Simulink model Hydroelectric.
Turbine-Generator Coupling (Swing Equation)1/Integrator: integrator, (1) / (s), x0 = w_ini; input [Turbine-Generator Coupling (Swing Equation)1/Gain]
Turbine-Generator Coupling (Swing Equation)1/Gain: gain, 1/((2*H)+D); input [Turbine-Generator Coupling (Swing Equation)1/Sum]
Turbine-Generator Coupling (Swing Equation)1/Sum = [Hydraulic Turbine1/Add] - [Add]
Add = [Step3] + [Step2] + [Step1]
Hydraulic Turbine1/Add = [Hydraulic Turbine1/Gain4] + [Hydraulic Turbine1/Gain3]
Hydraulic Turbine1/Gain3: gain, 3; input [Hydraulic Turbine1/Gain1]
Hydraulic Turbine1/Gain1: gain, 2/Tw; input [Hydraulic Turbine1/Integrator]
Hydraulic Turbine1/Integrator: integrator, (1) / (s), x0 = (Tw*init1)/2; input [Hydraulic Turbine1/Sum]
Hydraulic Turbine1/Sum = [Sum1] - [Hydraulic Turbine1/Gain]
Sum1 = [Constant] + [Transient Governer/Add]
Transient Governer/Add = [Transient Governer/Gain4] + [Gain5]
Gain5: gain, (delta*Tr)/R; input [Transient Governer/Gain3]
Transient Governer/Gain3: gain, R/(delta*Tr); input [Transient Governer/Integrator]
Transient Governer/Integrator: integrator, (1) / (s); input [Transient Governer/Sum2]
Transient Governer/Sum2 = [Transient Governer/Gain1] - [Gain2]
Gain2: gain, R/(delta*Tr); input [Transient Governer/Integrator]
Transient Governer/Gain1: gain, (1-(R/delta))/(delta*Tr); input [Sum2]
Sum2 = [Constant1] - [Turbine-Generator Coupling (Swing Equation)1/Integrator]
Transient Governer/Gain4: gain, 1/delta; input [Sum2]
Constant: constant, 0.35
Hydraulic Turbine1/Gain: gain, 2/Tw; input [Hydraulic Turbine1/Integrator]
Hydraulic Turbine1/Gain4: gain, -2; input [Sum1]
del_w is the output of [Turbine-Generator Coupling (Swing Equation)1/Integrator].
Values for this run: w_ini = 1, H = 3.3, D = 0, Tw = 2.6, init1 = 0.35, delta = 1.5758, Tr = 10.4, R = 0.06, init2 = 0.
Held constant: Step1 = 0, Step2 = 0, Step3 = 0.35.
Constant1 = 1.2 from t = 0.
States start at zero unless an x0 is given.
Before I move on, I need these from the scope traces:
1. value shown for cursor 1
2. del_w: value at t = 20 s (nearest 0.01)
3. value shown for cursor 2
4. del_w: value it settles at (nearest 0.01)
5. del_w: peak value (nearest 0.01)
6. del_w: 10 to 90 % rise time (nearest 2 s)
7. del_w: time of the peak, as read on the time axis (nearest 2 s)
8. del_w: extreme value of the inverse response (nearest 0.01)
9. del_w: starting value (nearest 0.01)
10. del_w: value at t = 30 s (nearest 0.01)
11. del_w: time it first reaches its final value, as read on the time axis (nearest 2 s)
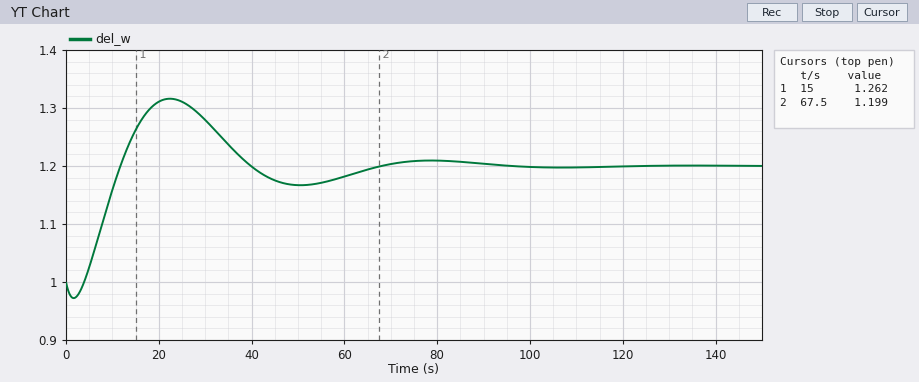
1.262
1.31
1.199
1.20
1.32
6 s
22 s
0.97
1.00
1.28
12 s
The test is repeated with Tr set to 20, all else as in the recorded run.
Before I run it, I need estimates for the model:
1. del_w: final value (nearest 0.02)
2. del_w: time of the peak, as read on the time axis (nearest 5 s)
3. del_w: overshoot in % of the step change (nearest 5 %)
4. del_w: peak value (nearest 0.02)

1.20
25 s
35 %
1.26
